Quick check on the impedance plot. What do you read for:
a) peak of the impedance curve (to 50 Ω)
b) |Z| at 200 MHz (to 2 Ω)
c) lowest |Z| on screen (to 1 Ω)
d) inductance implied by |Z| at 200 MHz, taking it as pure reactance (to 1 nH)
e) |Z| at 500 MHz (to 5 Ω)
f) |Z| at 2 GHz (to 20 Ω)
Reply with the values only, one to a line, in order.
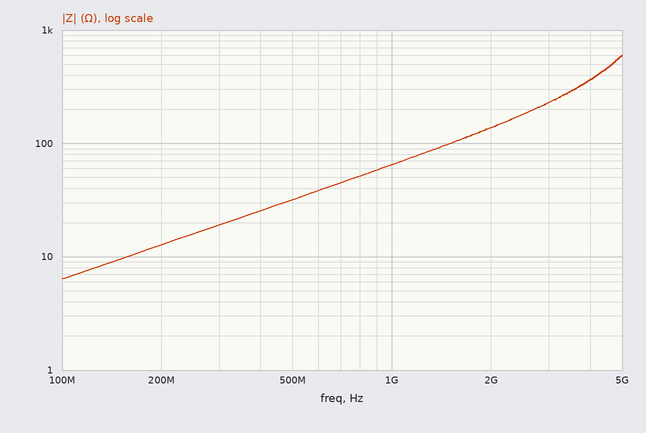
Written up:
600 Ω
12 Ω
6 Ω
10 nH
30 Ω
140 Ω
